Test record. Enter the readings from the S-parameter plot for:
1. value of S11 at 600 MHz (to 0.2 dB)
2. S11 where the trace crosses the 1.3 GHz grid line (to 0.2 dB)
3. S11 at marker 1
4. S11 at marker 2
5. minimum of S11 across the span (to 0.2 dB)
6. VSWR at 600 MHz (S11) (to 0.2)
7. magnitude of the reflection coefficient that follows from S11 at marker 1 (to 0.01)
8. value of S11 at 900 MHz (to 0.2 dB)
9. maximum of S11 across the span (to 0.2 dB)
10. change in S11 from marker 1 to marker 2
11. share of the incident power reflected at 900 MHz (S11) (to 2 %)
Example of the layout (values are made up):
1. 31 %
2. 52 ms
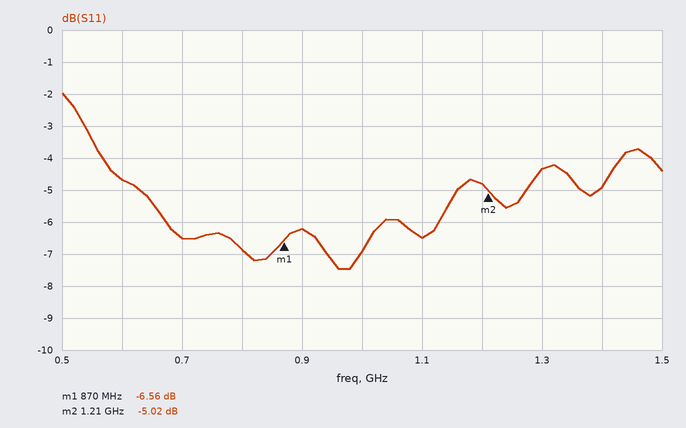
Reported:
1. -4.6 dB
2. -4.4 dB
3. -6.56 dB
4. -5.02 dB
5. -7.4 dB
6. 3.8
7. 0.47
8. -6.2 dB
9. -2.0 dB
10. 1.54 dB
11. 24 %
